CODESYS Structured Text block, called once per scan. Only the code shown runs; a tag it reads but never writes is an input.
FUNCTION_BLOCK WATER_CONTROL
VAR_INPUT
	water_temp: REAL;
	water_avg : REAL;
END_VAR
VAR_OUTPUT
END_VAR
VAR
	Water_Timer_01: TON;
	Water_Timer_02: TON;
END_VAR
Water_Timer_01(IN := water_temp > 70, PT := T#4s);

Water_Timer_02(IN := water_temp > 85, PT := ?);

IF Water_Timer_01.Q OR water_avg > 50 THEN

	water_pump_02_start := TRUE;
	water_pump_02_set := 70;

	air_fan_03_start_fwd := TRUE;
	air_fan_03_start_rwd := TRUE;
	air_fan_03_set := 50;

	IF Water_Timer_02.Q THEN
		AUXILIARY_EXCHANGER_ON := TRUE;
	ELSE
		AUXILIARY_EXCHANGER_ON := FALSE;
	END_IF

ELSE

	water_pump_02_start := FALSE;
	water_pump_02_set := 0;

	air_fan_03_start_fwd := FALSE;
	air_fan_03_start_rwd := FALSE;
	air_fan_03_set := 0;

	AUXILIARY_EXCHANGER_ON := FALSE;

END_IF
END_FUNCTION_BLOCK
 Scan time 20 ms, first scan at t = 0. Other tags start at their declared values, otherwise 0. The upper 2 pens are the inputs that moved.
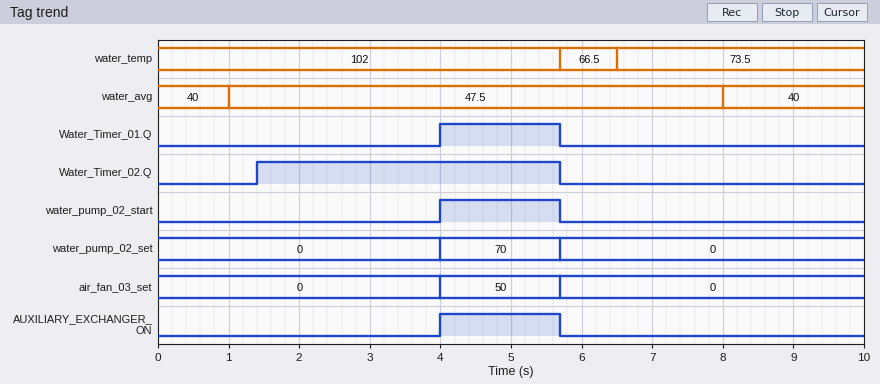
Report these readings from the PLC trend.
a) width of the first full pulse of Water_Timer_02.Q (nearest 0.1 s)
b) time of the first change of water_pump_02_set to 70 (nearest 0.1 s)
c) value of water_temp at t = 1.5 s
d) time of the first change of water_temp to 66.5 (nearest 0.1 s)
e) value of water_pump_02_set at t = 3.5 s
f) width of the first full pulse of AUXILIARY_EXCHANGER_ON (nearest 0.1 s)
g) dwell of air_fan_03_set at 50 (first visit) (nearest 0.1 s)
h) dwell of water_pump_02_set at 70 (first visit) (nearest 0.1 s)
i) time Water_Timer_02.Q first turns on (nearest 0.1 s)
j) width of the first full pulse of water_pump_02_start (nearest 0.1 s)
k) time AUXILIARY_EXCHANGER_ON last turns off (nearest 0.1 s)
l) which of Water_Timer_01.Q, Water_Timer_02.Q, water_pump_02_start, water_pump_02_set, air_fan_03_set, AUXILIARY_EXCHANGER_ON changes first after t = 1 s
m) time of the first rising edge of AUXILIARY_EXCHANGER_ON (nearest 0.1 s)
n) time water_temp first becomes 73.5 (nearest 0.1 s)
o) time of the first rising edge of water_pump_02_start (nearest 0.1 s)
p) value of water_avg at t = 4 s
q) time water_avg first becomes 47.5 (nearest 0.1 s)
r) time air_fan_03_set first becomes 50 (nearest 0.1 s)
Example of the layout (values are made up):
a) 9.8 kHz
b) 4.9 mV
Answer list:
a) 4.3 s
b) 4.0 s
c) 102
d) 5.7 s
e) 0
f) 1.7 s
g) 1.7 s
h) 1.7 s
i) 1.4 s
j) 1.7 s
k) 5.7 s
l) Water_Timer_02.Q
m) 4.0 s
n) 6.5 s
o) 4.0 s
p) 47.5
q) 1.0 s
r) 4.0 s
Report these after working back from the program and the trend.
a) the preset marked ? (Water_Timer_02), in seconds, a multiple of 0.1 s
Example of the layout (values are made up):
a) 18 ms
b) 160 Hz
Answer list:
a) 1.4 s
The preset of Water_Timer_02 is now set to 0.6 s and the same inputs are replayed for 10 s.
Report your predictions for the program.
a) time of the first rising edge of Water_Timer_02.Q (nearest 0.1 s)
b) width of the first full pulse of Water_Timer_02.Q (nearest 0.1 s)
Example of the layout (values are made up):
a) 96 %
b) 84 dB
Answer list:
a) 0.6 s
b) 5.1 s
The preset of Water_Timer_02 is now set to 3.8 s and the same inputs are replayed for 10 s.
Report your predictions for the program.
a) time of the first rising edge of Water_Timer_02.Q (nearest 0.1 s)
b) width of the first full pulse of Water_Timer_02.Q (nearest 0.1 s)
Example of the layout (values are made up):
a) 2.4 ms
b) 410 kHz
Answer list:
a) 3.8 s
b) 1.9 s
